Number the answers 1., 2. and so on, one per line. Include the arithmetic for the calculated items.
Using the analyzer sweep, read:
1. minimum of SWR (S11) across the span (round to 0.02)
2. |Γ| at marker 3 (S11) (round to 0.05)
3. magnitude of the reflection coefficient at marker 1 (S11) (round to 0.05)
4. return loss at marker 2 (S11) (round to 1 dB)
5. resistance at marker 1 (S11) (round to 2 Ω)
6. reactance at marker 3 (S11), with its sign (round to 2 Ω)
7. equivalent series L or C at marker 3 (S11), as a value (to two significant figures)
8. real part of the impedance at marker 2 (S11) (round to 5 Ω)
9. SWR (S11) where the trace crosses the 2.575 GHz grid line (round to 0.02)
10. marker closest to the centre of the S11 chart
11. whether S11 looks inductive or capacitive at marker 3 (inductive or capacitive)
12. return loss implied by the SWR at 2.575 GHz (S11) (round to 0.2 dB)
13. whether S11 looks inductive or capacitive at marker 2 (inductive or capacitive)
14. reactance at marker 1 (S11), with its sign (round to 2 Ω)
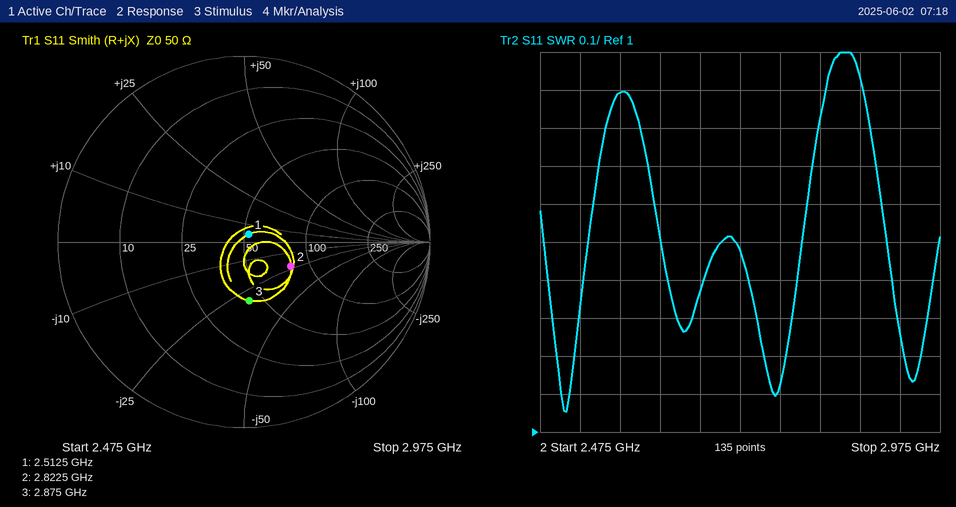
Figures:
1. 1.06
2. 0.30
3. 0.05
4. 11 dB
5. 52 Ω
6. -30 Ω
7. C = 1/(2π × 2.875 GHz × 30 Ω) ≈ 1.8 pF
8. 80 Ω
9. 1.90
10. marker 1
11. capacitive
12. −20 log10((1.9 − 1)/(1.9 + 1)) ≈ 10.2 dB
13. capacitive
14. +4 Ω
